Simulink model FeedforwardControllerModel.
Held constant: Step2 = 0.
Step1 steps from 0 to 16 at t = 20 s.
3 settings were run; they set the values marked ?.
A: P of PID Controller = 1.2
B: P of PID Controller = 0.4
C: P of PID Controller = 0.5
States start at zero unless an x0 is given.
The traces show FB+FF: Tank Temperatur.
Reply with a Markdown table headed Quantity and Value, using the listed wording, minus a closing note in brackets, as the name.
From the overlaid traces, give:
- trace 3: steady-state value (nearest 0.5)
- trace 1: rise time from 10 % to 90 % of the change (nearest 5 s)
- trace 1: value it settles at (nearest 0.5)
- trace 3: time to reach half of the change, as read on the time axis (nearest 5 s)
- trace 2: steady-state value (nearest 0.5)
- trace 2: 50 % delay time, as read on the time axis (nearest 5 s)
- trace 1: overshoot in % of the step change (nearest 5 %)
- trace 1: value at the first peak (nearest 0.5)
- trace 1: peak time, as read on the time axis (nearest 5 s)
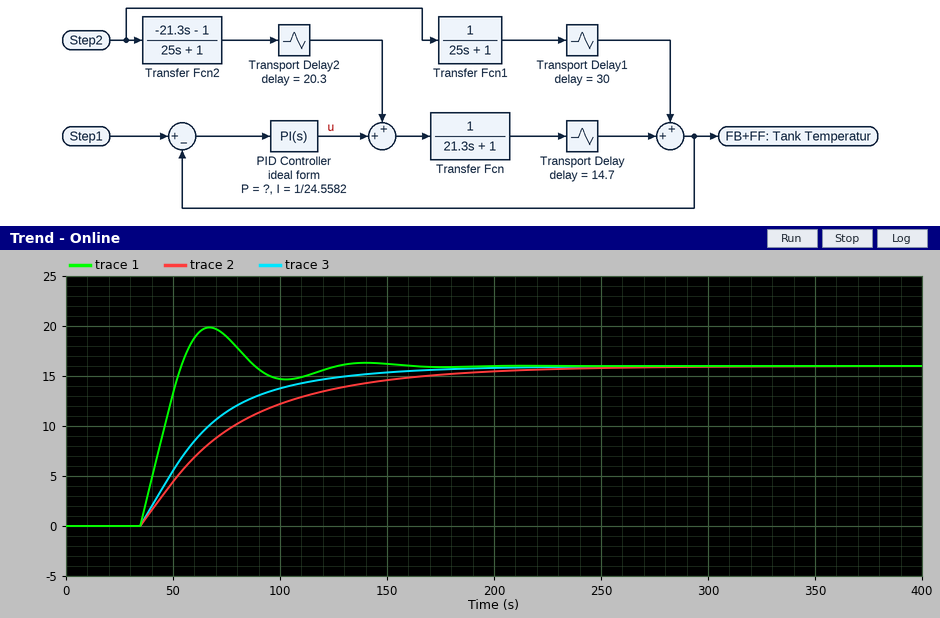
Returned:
| Quantity | Value |
|---|---|
| trace 3: steady-state value | 16.0 |
| trace 1: rise time from 10 % to 90 % of the change | 15 s |
| trace 1: value it settles at | 16.0 |
| trace 3: time to reach half of the change, as read on the time axis | 60 s |
| trace 2: steady-state value | 16.0 |
| trace 2: 50 % delay time, as read on the time axis | 65 s |
| trace 1: overshoot in % of the step change | 25 % |
| trace 1: value at the first peak | 20.0 |
| trace 1: peak time, as read on the time axis | 65 s |
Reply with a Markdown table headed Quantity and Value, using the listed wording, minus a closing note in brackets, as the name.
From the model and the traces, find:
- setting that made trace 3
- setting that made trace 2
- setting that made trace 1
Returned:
| Quantity | Value |
|---|---|
| setting that made trace 3 | C |
| setting that made trace 2 | B |
| setting that made trace 1 | A |
